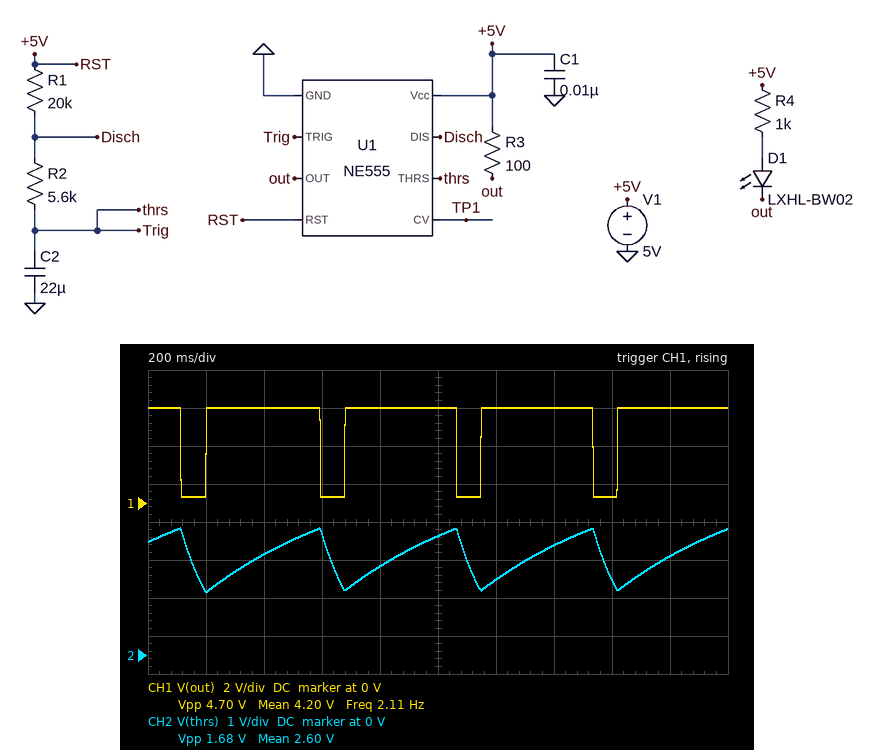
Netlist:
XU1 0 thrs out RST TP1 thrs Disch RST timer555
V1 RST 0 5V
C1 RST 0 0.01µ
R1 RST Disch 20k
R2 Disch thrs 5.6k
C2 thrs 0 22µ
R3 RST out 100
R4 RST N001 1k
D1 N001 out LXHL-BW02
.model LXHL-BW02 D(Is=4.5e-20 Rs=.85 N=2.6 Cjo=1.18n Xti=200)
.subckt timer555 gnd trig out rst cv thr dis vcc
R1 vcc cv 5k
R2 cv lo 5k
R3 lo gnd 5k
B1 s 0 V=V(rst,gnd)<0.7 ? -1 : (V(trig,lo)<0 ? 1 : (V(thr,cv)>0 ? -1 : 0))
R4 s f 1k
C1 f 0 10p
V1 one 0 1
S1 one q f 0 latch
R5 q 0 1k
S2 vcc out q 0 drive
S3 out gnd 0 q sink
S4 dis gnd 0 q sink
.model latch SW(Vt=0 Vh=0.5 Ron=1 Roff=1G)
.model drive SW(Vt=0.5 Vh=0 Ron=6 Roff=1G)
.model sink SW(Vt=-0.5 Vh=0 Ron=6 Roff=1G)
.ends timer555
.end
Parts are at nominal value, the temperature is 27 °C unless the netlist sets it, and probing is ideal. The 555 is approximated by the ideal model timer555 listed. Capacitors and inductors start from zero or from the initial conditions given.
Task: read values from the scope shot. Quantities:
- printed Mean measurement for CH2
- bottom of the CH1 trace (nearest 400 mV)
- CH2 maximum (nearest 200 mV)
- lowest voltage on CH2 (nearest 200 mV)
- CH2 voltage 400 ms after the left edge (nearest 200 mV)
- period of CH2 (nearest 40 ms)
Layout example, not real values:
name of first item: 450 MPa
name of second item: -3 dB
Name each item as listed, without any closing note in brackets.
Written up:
printed Mean measurement for CH2: 2.60 V
bottom of the CH1 trace: 400 mV
CH2 maximum: 3.4 V
lowest voltage on CH2: 1.6 V
CH2 voltage 400 ms after the left edge: 2.6 V
period of CH2: 480 ms
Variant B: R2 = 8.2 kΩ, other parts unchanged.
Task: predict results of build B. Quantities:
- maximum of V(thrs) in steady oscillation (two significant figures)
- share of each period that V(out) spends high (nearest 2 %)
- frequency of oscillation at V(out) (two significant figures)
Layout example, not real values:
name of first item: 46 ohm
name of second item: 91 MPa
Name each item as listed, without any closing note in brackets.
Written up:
maximum of V(thrs) in steady oscillation: 3.3 V
share of each period that V(out) spends high: 78 %
frequency of oscillation at V(out): 1.8 Hz
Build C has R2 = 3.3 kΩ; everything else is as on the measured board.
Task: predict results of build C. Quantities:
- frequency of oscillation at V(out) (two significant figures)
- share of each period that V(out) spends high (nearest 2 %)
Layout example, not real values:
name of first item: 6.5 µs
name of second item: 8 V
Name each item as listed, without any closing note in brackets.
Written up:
frequency of oscillation at V(out): 2.5 Hz
share of each period that V(out) spends high: 88 %
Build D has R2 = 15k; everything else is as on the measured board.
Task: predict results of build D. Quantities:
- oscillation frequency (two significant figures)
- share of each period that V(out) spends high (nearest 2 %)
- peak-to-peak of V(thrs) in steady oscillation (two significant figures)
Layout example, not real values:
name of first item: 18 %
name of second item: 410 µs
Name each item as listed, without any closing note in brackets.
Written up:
oscillation frequency: 1.3 Hz
share of each period that V(out) spends high: 70 %
peak-to-peak of V(thrs) in steady oscillation: 1.7 V
